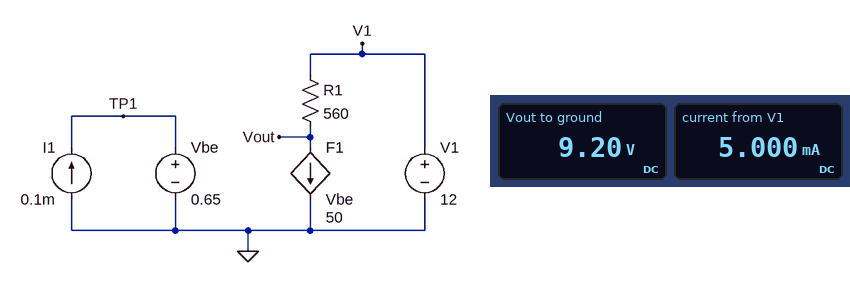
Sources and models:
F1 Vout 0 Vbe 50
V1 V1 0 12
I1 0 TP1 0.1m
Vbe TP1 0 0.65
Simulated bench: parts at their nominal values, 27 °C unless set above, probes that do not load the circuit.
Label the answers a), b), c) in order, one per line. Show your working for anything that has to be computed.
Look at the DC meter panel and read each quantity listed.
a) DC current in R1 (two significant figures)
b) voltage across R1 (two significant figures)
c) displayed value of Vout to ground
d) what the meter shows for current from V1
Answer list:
a) (12 V - 9.2 V) / 560 Ω = 5.0 mA
b) 12 V - 9.2 V = 2.8 V
c) 9.20 V
d) 5.000 mA
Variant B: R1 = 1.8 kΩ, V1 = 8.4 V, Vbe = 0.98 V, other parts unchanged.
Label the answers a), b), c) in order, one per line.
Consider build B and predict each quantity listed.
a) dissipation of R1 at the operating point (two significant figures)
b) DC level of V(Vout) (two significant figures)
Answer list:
a) 45 mW
b) -600 mV
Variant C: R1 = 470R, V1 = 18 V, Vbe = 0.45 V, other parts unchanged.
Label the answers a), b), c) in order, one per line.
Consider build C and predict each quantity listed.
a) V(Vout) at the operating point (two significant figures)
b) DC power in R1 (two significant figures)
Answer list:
a) 16 V
b) 12 mW
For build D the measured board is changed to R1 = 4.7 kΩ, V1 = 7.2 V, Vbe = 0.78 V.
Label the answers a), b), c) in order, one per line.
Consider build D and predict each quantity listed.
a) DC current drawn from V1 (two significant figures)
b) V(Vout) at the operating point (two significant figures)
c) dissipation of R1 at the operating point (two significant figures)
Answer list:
a) 5.0 mA
b) -16 V
c) 120 mW
